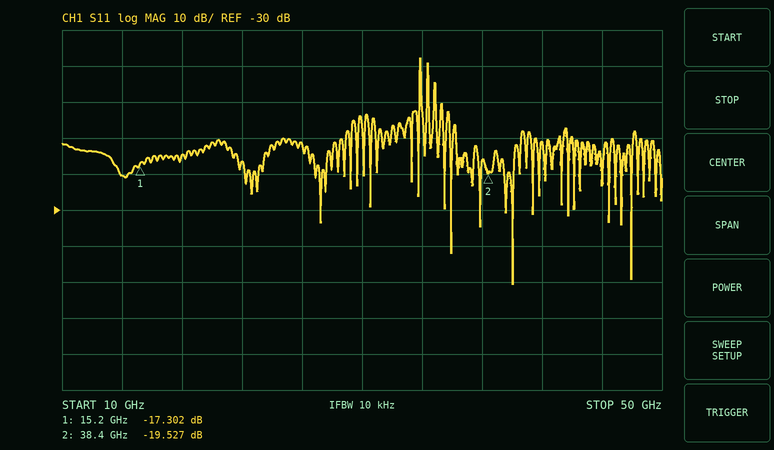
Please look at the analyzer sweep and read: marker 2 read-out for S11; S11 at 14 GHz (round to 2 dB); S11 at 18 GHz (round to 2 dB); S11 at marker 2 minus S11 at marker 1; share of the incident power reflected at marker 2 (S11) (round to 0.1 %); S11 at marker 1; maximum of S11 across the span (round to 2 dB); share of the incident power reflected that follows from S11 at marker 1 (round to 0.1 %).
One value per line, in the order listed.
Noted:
-19.527 dB
-20 dB
-14 dB
-2.225 dB
1.1 %
-17.302 dB
12 dB
1.9 %
